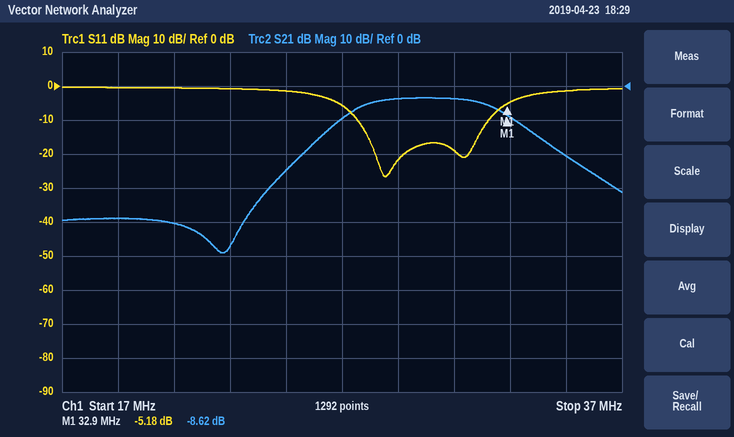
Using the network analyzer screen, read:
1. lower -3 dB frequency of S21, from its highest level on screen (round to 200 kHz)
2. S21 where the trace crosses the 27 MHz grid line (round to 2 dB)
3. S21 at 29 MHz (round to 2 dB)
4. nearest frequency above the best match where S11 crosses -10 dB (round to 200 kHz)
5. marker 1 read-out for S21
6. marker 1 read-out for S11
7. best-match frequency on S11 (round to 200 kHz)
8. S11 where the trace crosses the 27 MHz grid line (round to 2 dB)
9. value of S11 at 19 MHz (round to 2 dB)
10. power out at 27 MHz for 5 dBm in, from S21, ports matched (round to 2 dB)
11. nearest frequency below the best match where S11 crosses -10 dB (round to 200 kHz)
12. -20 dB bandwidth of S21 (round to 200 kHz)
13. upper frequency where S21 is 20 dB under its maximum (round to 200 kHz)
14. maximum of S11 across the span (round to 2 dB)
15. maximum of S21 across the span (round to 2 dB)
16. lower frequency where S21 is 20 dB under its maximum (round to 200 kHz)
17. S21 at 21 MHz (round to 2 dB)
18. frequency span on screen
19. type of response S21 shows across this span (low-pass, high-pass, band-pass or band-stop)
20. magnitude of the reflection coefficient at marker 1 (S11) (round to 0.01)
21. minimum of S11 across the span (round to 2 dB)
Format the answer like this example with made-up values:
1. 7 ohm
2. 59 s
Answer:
1. 27.6 MHz
2. -10 dB
3. -4 dB
4. 32.2 MHz
5. -8.62 dB
6. -5.18 dB
7. 28.6 MHz
8. -6 dB
9. 0 dB
10. -4 dBm
11. 27.6 MHz
12. 10.4 MHz
13. 35.6 MHz
14. 0 dB
15. -4 dB
16. 25.2 MHz
17. -40 dB
18. 20 MHz
19. band-pass
20. 0.55
21. -26 dB
